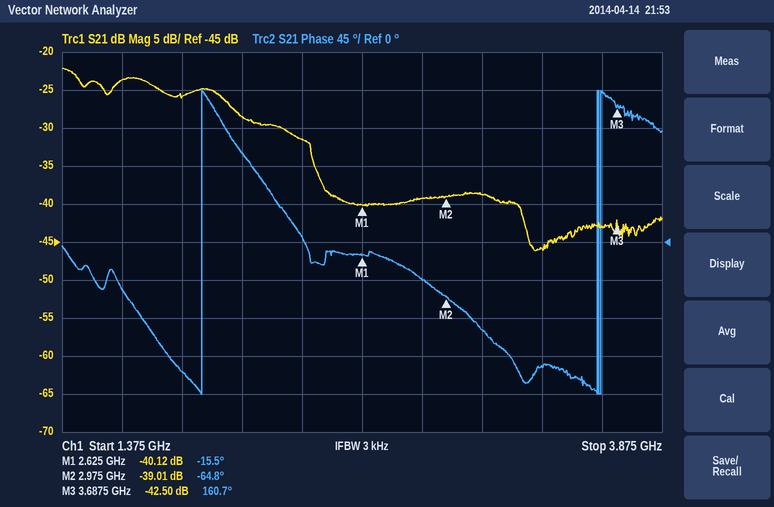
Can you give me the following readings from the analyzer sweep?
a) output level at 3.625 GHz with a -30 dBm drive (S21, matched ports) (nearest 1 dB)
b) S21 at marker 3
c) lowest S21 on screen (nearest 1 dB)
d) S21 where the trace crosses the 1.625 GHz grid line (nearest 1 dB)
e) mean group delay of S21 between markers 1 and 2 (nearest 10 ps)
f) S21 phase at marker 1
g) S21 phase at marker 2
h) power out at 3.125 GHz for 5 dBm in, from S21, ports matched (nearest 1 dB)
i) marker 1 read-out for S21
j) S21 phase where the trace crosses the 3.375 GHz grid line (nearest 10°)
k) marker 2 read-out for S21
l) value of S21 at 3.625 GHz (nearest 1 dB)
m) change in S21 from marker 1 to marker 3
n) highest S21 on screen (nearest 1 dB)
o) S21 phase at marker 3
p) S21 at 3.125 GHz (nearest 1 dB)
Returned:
-73 dBm
-42.50 dB
-46 dB
-24 dB
390 ps
-15.5°
-64.8°
-34 dBm
-40.12 dB
-150°
-39.01 dB
-43 dB
-2.38 dB
-22 dB
160.7°
-39 dB
